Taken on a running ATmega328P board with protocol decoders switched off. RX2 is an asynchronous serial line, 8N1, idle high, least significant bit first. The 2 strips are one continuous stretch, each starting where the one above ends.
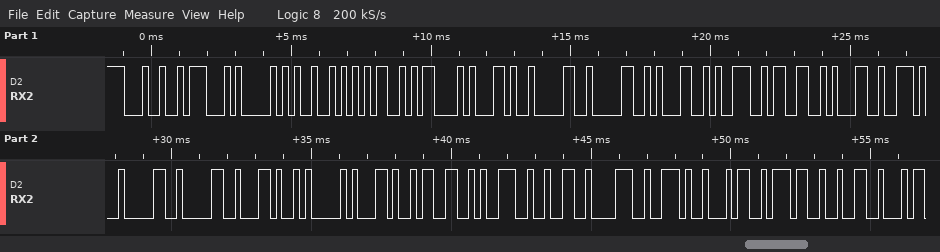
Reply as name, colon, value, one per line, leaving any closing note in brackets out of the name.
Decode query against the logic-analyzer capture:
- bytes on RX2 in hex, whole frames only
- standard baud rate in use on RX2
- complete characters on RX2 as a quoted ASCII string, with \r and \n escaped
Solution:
bytes on RX2 in hex, whole frames only: 0x24 0x47 0x50 0x52 0x4D 0x43 0x2C 0x30 0x30 0x31 0x39 0x33 0x31 0x2E 0x30 0x30 0x2C 0x41 0x2C 0x33 0x39 0x32 0x38 0x2E 0x34 0x37 0x32
standard baud rate in use on RX2: 4800 baud
complete characters on RX2 as a quoted ASCII string, with \r and \n escaped: "$GPRMC,001931.00,A,3928.472"
